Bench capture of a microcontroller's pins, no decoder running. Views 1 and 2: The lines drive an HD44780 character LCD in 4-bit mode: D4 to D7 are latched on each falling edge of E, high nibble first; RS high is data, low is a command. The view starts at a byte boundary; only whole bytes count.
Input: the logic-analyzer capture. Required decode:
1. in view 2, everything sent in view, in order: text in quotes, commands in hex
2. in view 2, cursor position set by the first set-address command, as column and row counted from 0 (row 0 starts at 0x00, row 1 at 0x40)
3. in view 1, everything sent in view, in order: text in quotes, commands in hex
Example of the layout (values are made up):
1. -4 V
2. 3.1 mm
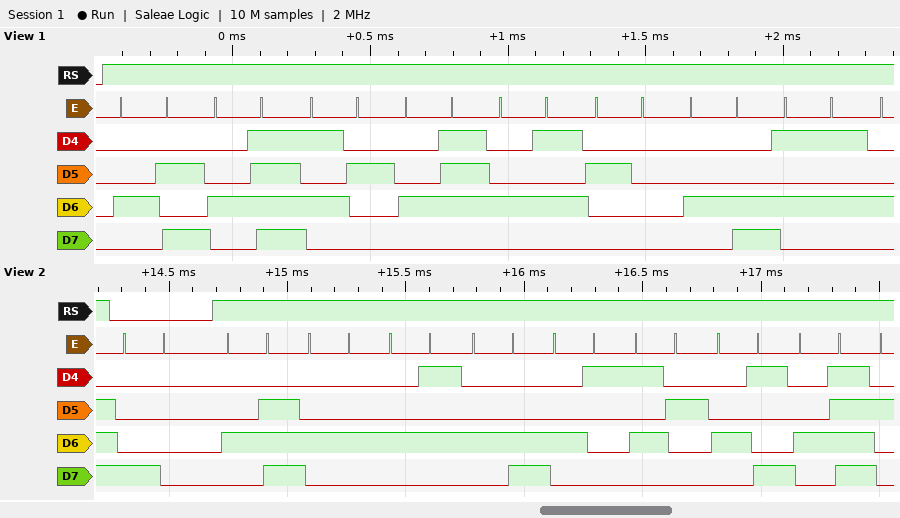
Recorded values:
1. 0x80 "NDELARIO"
2. column 0, row 0
3. "JORGE LU"
